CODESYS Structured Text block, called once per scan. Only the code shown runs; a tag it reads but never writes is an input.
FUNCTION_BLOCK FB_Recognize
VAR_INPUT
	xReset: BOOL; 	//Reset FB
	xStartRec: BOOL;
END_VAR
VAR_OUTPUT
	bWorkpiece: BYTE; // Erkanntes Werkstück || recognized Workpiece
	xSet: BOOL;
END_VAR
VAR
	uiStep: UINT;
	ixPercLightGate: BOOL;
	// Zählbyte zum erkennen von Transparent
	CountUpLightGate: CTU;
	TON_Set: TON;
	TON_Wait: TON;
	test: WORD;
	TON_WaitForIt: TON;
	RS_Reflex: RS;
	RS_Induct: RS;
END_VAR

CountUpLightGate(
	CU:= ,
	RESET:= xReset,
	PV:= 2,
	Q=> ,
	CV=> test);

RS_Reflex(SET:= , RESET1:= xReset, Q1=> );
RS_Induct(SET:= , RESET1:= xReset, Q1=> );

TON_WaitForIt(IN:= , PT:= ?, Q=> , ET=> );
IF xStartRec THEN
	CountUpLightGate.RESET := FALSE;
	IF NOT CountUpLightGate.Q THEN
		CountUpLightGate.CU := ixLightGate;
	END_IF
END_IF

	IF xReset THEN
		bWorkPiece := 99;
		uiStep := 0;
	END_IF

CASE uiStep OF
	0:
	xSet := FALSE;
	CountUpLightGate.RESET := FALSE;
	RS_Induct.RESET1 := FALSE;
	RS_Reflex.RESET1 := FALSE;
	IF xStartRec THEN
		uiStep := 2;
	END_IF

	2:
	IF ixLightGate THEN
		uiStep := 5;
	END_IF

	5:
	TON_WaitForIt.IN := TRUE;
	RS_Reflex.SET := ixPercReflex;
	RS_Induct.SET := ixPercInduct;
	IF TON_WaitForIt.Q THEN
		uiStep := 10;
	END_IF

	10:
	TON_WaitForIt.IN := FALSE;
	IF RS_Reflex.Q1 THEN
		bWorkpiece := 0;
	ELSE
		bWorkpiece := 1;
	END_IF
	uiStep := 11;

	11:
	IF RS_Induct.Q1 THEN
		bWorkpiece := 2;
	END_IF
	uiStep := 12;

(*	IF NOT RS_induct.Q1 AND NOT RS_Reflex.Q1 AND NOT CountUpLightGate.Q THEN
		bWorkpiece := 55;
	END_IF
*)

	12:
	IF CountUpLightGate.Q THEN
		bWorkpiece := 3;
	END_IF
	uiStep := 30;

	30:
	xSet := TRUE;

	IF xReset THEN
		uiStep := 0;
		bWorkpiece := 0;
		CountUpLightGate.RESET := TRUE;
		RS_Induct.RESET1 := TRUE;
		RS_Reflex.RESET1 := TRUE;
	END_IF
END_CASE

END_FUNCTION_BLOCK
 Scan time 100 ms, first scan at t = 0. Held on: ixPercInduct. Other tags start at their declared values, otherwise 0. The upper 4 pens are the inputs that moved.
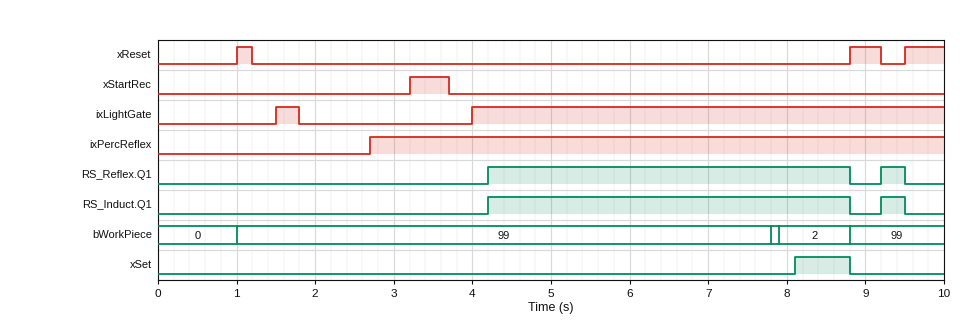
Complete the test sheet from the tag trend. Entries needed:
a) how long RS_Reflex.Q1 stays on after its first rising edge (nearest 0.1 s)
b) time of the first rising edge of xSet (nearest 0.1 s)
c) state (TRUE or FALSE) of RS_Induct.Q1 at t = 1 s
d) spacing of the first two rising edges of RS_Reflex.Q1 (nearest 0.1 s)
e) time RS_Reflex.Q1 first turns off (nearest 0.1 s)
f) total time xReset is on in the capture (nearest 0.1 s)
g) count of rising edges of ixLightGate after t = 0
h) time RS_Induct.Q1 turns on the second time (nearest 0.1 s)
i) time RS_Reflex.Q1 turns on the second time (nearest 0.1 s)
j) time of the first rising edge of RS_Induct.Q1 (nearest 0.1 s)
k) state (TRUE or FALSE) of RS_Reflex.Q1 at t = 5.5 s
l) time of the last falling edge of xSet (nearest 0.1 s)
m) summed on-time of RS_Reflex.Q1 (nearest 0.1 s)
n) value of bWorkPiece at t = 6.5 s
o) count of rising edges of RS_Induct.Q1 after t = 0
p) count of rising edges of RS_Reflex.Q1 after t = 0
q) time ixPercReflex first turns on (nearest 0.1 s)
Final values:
4.6 s
8.1 s
FALSE
5.0 s
8.8 s
1.1 s
2
9.2 s
9.2 s
4.2 s
TRUE
8.8 s
4.9 s
99
2
2
2.7 s
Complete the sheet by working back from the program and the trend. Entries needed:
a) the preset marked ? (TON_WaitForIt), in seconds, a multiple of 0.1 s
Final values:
3.5 s
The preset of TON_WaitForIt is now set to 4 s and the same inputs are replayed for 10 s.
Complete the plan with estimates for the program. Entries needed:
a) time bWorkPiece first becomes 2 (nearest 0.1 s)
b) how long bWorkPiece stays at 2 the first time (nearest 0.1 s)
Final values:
8.4 s
0.4 s
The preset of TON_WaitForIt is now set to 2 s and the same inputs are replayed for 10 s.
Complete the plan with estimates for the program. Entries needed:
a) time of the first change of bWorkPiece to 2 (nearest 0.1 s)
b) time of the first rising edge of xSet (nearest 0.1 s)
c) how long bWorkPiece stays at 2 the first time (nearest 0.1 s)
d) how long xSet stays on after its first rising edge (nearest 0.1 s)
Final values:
6.4 s
6.6 s
2.4 s
2.2 s
